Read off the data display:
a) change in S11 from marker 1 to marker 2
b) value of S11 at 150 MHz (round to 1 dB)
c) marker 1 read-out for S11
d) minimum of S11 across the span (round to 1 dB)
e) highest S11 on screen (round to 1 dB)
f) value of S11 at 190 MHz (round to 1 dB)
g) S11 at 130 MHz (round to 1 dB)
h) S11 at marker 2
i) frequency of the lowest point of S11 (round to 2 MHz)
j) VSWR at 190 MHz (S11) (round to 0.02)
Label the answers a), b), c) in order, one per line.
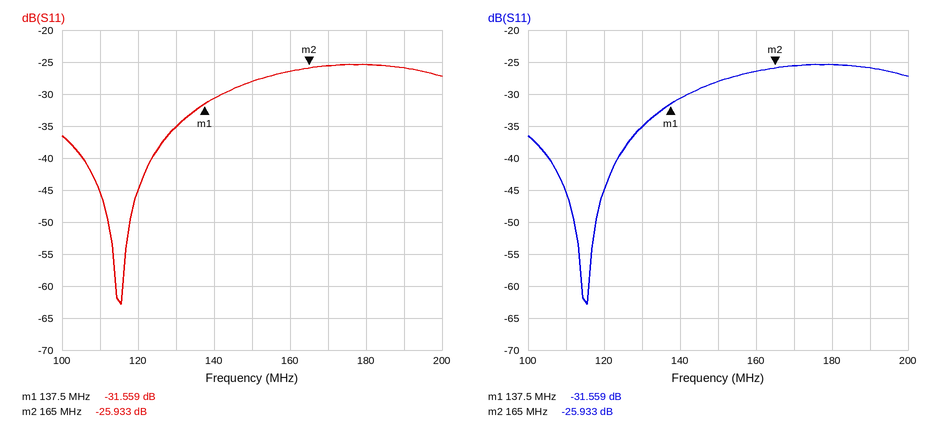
a) 5.626 dB
b) -28 dB
c) -31.559 dB
d) -63 dB
e) -25 dB
f) -26 dB
g) -35 dB
h) -25.933 dB
i) 116 MHz
j) 1.10
